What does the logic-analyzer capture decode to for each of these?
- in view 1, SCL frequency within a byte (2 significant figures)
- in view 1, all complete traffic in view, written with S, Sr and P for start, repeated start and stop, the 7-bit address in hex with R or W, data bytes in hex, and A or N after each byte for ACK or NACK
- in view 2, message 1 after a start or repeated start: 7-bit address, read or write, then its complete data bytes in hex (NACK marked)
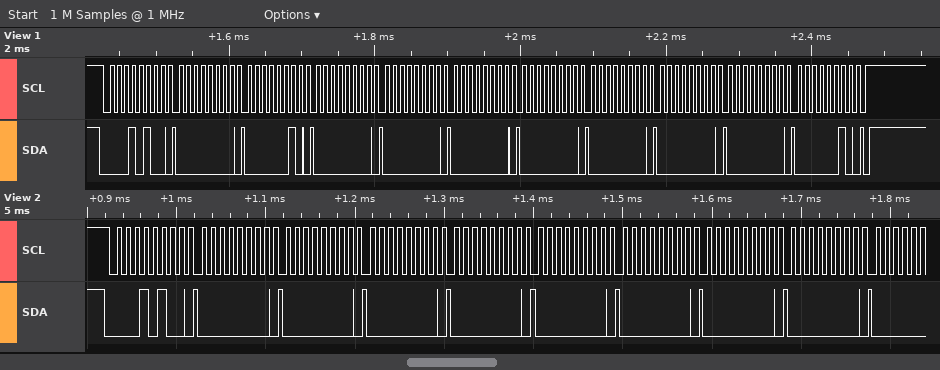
100 kHz
S 0AW A 00 A 02 A 00 A 00 A 00 A 00 A 00 A 00 A 00 A 02 A P
0x0A write: 00 00 00 00 00 00 00 00
